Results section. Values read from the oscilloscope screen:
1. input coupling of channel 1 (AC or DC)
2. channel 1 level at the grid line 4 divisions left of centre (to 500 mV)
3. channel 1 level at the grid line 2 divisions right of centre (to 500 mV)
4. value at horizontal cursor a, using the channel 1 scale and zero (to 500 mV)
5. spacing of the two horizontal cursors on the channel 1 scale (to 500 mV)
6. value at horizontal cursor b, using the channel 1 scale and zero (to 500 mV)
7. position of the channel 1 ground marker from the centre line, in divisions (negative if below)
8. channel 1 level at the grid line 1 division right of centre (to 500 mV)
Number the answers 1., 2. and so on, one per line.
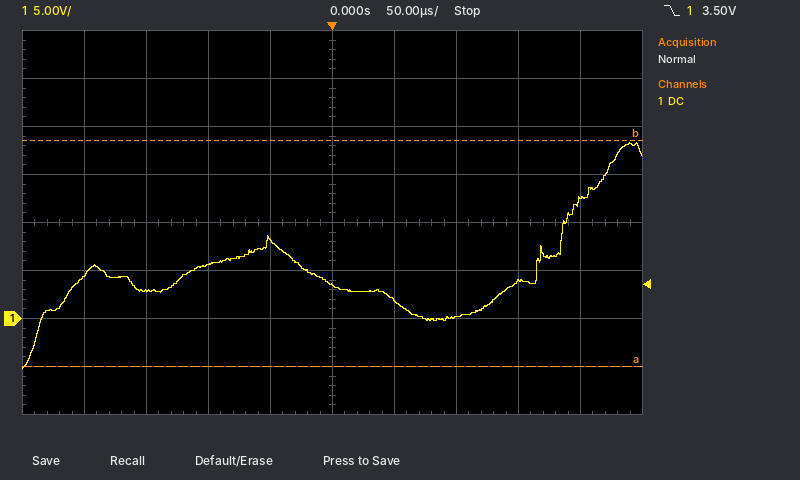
1. DC
2. 4.5 V
3. 0.0 V
4. -5.0 V
5. 23.5 V
6. 18.5 V
7. -2.0 div
8. 2.0 V
